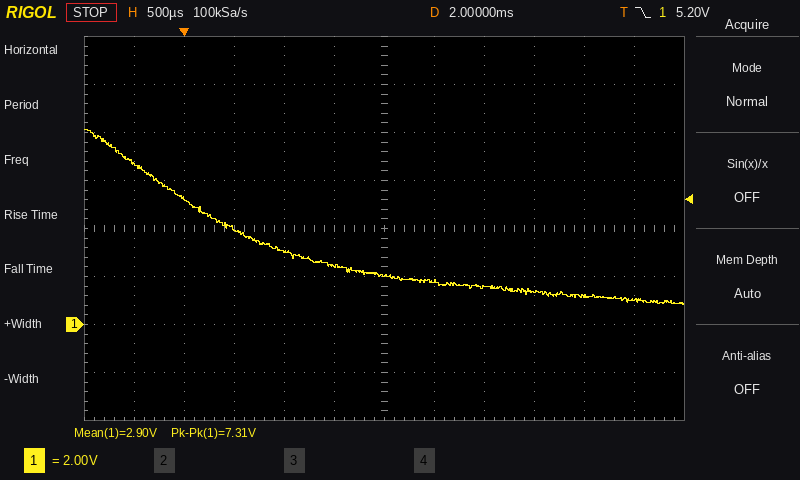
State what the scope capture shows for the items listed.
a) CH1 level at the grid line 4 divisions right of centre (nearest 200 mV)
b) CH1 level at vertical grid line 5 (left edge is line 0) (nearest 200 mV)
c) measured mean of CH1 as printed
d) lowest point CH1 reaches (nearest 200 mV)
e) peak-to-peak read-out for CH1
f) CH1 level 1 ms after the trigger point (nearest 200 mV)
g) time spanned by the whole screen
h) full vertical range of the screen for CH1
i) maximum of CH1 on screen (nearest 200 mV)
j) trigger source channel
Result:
1.2 V
2.4 V
2.90 V
800 mV
7.31 V
3.0 V
6 ms
16 V
8.2 V
CH1
